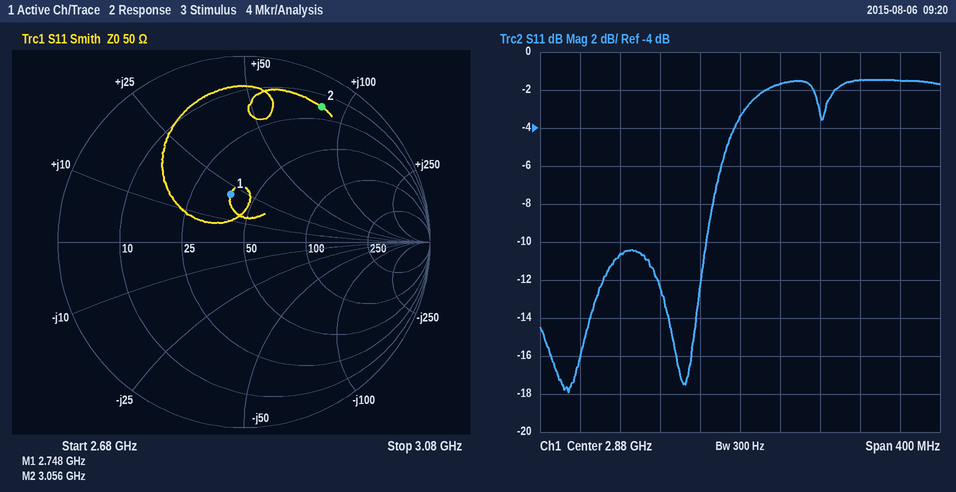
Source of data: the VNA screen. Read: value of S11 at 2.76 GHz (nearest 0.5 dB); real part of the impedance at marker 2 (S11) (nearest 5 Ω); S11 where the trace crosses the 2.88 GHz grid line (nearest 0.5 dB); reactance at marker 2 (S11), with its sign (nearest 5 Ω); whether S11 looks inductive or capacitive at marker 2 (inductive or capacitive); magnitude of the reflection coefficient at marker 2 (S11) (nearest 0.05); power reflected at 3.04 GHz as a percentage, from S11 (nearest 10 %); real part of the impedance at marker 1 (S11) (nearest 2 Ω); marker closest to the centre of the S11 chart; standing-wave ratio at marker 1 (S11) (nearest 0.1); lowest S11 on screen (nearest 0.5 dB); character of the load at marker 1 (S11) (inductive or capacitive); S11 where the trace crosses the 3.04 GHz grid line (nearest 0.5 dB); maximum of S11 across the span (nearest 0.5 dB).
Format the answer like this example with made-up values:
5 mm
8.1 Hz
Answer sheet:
-10.5 dB
15 Ω
-3.5 dB
+85 Ω
inductive
0.85
70 %
38 Ω
marker 1
1.7
-18.0 dB
inductive
-1.5 dB
-1.5 dB
